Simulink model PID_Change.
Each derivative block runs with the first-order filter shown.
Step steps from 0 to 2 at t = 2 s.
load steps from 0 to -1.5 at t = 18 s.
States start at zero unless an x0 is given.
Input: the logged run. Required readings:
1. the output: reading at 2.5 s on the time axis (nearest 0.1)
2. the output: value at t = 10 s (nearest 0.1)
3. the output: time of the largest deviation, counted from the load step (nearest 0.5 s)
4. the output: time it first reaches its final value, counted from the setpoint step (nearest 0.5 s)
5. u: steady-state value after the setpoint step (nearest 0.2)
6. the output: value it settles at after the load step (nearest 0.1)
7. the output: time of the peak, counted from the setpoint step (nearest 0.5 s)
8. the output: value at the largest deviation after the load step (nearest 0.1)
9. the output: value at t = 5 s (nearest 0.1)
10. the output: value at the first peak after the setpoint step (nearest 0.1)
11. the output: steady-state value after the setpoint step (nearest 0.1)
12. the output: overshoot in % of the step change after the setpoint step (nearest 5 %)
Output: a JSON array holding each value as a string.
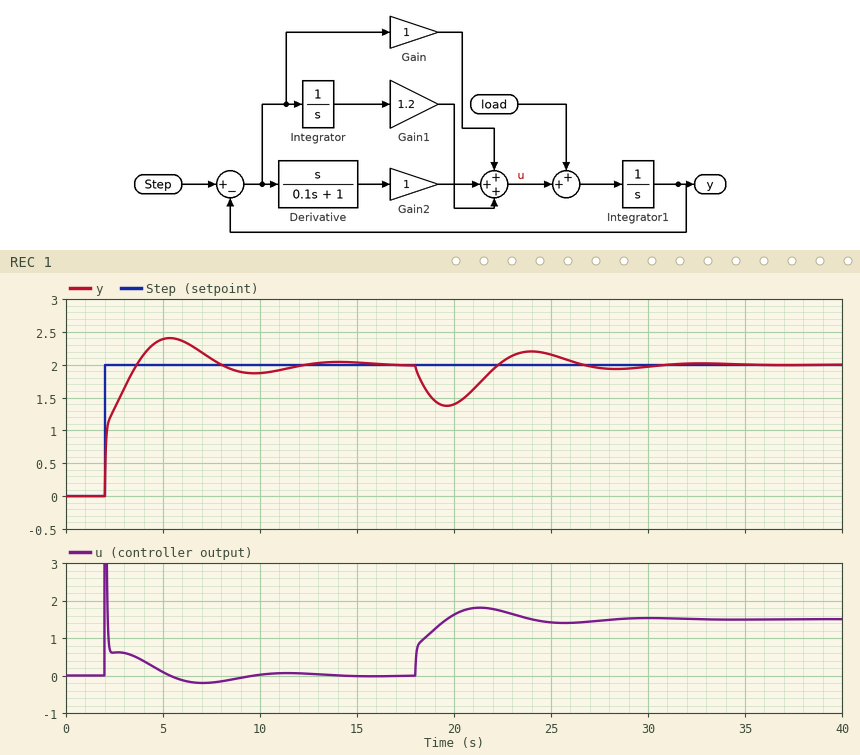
["1.3", "1.9", "1.5 s", "1.5 s", "0.0", "2.0", "3.5 s", "1.4", "2.4", "2.4", "2.0", "20 %"]
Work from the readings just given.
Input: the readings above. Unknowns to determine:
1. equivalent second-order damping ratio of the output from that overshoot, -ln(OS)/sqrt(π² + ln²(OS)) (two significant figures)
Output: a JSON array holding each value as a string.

["0.46"]
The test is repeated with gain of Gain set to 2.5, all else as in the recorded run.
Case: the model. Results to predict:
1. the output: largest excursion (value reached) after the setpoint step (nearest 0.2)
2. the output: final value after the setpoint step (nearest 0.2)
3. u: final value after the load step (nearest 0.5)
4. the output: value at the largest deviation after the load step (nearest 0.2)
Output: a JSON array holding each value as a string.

["2.2", "2.0", "1.5", "1.6"]
